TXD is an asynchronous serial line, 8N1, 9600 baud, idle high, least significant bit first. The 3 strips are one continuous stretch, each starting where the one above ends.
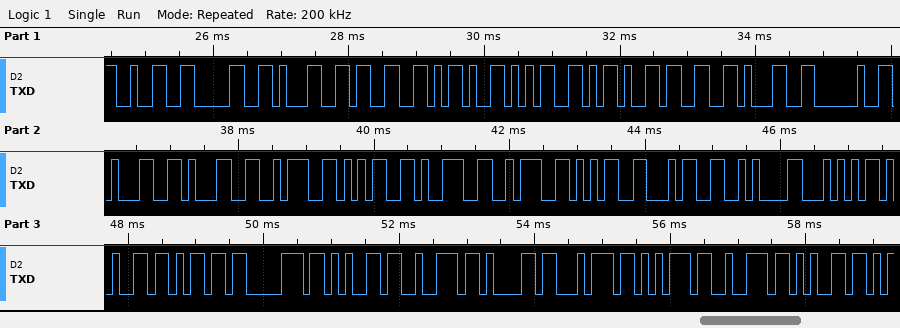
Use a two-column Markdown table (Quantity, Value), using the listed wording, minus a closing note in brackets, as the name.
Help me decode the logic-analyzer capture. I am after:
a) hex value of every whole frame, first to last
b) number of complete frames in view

| Quantity | Value |
|---|---|
| hex value of every whole frame, first to last | 32 30 31 33 2D 35 2D 33 31 20 31 31 3A 35 39 3A 35 34 0A 54 65 6D 70 65 72 61 74 75 72 65 |
| number of complete frames in view | 30 |
